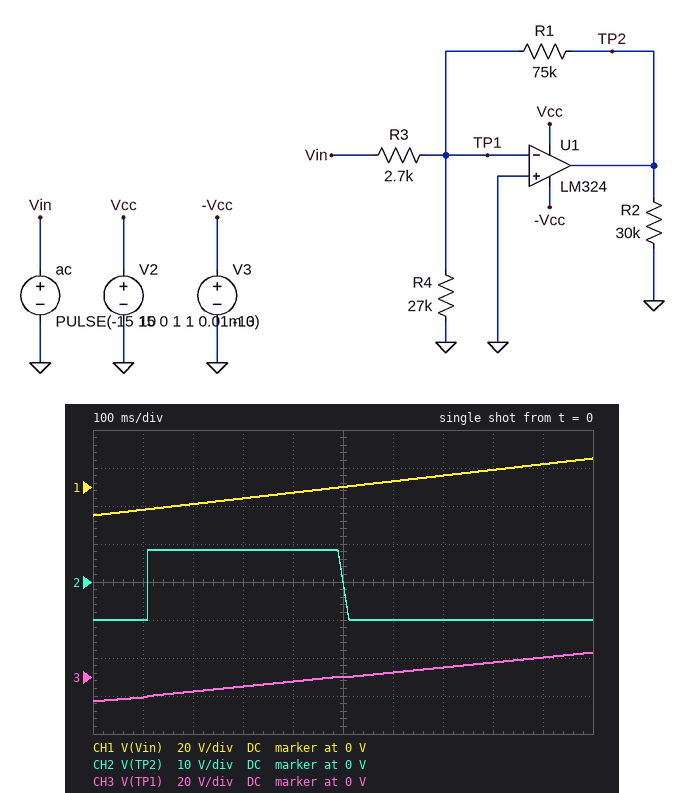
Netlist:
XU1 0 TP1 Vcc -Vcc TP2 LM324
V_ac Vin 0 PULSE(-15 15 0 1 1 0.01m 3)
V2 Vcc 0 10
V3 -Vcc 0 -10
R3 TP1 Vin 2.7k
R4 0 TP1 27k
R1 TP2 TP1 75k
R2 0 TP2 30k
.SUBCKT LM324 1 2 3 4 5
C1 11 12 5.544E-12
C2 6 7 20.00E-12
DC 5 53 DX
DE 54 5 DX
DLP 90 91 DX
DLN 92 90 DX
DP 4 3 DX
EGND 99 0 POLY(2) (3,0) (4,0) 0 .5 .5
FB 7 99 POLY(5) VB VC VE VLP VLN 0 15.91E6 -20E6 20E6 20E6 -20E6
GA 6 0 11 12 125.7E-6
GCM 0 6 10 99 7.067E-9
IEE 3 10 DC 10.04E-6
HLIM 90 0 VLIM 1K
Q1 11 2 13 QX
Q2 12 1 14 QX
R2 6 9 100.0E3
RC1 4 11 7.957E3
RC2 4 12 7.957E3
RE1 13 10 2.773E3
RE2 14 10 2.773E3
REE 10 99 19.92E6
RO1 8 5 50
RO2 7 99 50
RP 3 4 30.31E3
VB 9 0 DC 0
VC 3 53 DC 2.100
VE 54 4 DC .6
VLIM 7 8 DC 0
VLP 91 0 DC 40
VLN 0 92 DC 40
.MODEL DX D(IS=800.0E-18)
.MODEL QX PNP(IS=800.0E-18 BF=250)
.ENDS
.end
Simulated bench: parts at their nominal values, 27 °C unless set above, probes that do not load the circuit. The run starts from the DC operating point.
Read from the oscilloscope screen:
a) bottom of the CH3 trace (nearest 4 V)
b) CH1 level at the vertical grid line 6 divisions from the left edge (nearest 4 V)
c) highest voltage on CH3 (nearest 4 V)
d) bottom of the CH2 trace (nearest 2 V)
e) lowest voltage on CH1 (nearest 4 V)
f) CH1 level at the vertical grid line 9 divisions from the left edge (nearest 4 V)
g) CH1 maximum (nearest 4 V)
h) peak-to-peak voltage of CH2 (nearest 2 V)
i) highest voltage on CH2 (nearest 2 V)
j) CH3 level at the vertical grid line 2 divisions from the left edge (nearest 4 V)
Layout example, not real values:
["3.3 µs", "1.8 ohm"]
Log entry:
["-12 V", "4 V", "12 V", "-10 V", "-16 V", "12 V", "16 V", "18 V", "8 V", "-8 V"]
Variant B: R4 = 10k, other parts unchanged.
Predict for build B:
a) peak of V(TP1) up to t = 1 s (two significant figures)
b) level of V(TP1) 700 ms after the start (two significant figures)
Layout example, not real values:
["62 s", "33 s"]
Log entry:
["11 V", "4.3 V"]
